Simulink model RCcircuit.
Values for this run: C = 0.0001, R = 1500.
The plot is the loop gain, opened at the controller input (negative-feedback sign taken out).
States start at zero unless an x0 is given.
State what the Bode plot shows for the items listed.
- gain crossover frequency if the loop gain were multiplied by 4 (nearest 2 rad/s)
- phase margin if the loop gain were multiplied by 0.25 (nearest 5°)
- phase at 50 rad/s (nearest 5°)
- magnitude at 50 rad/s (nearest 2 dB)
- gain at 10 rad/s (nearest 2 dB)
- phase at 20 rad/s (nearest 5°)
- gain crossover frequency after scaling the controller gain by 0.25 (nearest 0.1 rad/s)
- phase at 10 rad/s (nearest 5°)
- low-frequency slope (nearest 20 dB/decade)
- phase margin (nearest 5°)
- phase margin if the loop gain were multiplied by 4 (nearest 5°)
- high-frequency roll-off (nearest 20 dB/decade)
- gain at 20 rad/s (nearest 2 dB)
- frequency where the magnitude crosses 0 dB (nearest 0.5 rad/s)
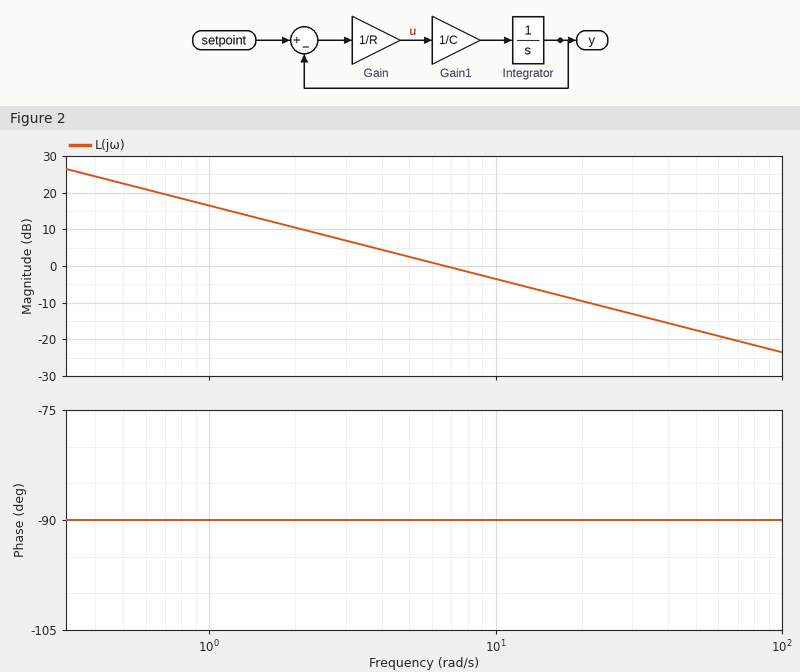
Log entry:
26 rad/s
90°
-90°
-18 dB
-4 dB
-90°
1.7 rad/s
-90°
-20 dB/decade
90°
90°
-20 dB/decade
-10 dB
6.5 rad/s
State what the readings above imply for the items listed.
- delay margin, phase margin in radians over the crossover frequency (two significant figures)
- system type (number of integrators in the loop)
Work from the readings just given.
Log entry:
0.24 s
1
